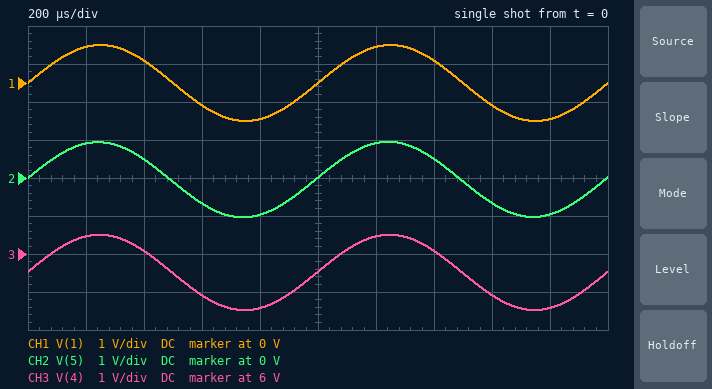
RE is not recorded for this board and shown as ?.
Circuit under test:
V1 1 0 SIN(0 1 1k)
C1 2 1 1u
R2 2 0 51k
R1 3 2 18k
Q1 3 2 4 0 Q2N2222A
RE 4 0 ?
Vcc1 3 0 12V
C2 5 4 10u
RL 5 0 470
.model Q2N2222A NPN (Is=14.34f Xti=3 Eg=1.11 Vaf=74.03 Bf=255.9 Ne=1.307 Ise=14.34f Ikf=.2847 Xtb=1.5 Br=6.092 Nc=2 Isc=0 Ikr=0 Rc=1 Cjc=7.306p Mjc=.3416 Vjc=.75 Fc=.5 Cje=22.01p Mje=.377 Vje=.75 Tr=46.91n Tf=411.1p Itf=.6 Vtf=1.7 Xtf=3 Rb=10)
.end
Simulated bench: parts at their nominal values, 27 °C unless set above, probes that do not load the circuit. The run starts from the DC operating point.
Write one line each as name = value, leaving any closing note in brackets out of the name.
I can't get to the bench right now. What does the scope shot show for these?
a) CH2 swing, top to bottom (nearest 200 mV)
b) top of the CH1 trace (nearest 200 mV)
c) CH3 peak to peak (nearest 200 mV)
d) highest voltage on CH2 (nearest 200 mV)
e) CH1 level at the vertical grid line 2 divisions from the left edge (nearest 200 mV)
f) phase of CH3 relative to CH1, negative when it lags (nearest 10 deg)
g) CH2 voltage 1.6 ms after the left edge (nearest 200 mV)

CH2 swing, top to bottom = 2.0 V
top of the CH1 trace = 1.0 V
CH3 peak to peak = 2.0 V
highest voltage on CH2 = 1.0 V
CH1 level at the vertical grid line 2 divisions from the left edge = 600 mV
phase of CH3 relative to CH1, negative when it lags = 0 deg
CH2 voltage 1.6 ms after the left edge = -600 mV
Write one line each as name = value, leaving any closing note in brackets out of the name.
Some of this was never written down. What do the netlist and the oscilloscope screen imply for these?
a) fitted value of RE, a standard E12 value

fitted value of RE, a standard E12 value = 150 Ω
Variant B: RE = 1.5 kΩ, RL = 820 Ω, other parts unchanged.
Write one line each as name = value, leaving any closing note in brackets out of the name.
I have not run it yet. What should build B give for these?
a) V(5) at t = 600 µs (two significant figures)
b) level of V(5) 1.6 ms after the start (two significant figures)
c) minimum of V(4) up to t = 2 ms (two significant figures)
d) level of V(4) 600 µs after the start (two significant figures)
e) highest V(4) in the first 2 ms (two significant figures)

V(5) at t = 600 µs = -640 mV
level of V(5) 1.6 ms after the start = -630 mV
minimum of V(4) up to t = 2 ms = 6.8 V
level of V(4) 600 µs after the start = 7.2 V
highest V(4) in the first 2 ms = 8.8 V
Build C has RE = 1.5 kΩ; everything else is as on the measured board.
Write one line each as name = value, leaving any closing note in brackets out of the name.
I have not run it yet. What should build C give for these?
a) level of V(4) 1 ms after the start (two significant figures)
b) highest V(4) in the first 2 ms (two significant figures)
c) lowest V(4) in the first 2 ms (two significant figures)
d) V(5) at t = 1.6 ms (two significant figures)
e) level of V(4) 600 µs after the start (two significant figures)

level of V(4) 1 ms after the start = 7.8 V
highest V(4) in the first 2 ms = 8.8 V
lowest V(4) in the first 2 ms = 6.8 V
V(5) at t = 1.6 ms = -650 mV
level of V(4) 600 µs after the start = 7.2 V
